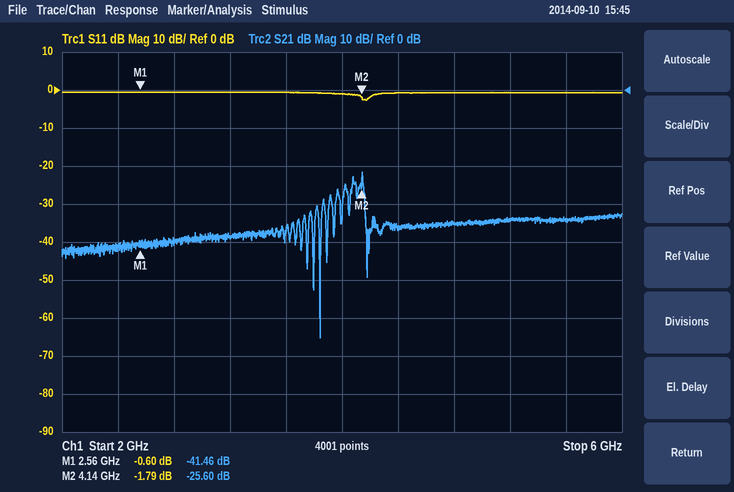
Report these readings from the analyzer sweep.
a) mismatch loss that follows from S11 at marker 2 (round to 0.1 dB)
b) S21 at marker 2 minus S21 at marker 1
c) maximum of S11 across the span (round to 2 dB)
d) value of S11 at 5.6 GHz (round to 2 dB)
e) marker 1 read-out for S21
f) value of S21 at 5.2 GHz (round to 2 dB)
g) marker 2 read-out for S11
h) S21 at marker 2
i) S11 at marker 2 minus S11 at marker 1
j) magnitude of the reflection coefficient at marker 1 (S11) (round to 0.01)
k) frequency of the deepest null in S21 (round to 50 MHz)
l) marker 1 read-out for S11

4.7 dB
15.86 dB
0 dB
0 dB
-41.46 dB
-34 dB
-1.79 dB
-25.60 dB
-1.19 dB
0.93
3.85 GHz
-0.60 dB
